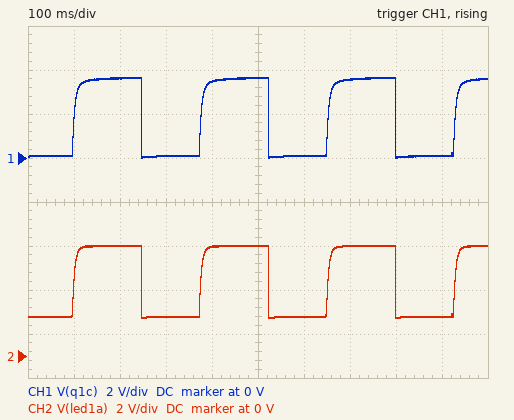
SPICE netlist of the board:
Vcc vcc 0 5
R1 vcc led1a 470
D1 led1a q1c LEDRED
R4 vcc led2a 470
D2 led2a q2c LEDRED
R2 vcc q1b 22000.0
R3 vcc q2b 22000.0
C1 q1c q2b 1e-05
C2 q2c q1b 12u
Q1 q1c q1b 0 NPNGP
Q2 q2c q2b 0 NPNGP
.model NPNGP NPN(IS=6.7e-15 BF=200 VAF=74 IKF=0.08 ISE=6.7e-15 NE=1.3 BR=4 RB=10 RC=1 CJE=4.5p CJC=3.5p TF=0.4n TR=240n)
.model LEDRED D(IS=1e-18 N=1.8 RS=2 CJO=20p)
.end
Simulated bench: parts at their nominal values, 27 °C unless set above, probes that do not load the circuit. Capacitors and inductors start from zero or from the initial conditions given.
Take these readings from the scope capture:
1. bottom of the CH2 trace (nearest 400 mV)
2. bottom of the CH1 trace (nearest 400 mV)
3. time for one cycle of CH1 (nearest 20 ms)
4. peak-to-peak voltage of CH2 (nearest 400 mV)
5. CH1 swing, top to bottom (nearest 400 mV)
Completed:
1.6 V
0 V
280 ms
3.2 V
3.6 V
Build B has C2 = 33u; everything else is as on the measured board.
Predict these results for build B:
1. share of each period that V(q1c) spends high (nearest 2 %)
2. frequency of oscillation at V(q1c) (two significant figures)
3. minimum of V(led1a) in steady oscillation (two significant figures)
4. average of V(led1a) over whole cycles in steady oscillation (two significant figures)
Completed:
76 %
1.9 Hz
1.7 V
4.2 V
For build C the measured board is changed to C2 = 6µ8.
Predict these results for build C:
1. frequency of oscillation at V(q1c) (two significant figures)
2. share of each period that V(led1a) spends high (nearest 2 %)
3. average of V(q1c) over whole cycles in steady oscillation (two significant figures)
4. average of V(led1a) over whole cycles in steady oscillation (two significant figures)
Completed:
4.7 Hz
40 %
1.4 V
3.0 V
